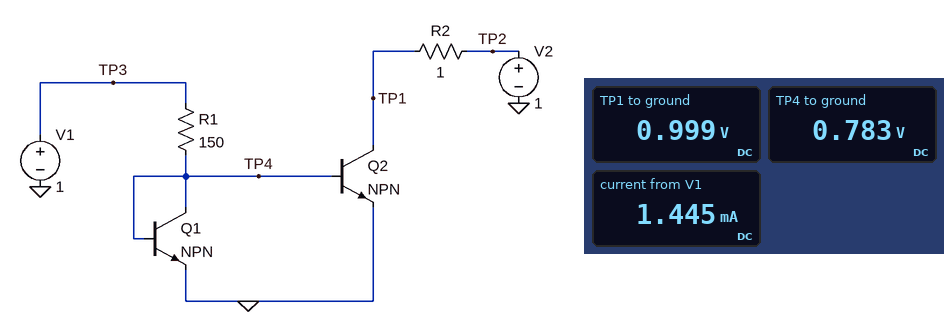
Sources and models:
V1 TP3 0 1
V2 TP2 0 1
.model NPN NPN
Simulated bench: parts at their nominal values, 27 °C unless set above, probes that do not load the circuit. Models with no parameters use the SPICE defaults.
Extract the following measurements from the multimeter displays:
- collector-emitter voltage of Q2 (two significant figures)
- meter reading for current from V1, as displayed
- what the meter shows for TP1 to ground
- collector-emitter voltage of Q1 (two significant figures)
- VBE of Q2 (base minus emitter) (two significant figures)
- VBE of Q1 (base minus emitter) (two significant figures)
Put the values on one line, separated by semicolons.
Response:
1.0 V; 1.445 mA; 0.999 V; 780 mV; 780 mV; 780 mV
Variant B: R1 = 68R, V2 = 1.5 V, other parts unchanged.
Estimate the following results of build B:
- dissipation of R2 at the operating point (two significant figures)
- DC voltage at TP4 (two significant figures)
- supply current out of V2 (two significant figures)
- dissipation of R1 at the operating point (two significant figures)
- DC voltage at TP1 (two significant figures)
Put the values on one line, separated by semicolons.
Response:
8.2 µW; 800 mV; 2.9 mA; 580 µW; 1.5 V
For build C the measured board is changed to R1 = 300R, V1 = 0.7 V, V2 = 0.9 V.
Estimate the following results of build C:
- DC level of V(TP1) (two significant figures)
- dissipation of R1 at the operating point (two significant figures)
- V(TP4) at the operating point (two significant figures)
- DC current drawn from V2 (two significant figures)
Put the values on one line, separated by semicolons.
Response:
900 mV; 420 nW; 690 mV; 37 µA
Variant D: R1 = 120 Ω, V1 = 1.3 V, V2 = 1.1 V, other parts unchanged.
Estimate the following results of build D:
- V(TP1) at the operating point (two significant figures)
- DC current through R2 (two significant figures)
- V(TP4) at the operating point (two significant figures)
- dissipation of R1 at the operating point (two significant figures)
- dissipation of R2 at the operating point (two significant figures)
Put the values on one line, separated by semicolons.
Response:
1.1 V; 4.0 mA; 810 mV; 2.0 mW; 16 µW
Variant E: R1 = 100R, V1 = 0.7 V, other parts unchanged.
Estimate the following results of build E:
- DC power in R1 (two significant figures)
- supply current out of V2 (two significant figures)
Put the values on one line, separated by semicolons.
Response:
230 nW; 47 µA
